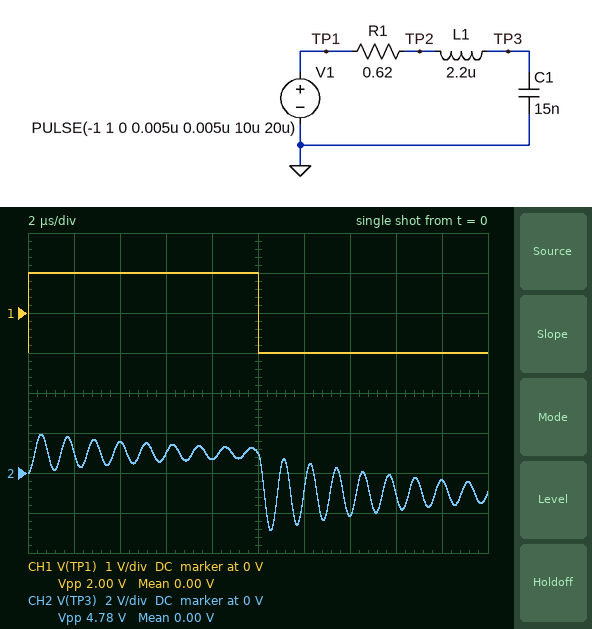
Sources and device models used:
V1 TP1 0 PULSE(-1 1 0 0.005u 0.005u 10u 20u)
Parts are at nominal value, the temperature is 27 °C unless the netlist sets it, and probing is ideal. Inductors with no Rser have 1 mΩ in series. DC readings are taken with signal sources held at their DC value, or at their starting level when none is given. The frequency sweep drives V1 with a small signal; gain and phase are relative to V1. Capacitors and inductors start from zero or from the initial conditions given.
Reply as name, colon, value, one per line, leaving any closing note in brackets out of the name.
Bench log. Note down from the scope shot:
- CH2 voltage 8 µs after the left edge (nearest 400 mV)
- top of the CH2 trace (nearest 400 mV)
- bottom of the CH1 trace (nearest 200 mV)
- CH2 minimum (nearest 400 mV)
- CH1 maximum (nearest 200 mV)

CH2 voltage 8 µs after the left edge: 800 mV
top of the CH2 trace: 2.0 V
bottom of the CH1 trace: -1.0 V
CH2 minimum: -2.8 V
CH1 maximum: 1.0 V
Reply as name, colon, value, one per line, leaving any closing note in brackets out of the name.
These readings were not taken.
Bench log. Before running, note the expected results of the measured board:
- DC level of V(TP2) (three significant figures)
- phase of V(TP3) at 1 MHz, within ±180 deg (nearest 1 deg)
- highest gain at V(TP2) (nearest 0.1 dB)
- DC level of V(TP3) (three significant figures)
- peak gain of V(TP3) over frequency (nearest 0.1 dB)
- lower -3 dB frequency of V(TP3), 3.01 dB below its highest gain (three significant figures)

DC level of V(TP2): -1.00 V
phase of V(TP3) at 1 MHz, within ±180 deg: -169 deg
highest gain at V(TP2): 0 dB
DC level of V(TP3): -1.00 V
peak gain of V(TP3) over frequency: 25.8 dB
lower -3 dB frequency of V(TP3), 3.01 dB below its highest gain: 853 kHz
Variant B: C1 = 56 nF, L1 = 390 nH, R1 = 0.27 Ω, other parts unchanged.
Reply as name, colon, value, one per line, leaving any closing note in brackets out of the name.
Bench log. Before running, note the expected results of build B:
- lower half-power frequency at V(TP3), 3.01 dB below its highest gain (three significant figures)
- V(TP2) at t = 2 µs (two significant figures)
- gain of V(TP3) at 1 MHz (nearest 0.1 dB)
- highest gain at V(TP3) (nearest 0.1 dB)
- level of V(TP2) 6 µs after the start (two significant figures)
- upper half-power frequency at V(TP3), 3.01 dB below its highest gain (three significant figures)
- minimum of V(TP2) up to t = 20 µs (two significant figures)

lower half-power frequency at V(TP3), 3.01 dB below its highest gain: 1.02 MHz
V(TP2) at t = 2 µs: 960 mV
gain of V(TP3) at 1 MHz: 15.5 dB
highest gain at V(TP3): 19.8 dB
level of V(TP2) 6 µs after the start: 1.0 V
upper half-power frequency at V(TP3), 3.01 dB below its highest gain: 1.13 MHz
minimum of V(TP2) up to t = 20 µs: -1.2 V
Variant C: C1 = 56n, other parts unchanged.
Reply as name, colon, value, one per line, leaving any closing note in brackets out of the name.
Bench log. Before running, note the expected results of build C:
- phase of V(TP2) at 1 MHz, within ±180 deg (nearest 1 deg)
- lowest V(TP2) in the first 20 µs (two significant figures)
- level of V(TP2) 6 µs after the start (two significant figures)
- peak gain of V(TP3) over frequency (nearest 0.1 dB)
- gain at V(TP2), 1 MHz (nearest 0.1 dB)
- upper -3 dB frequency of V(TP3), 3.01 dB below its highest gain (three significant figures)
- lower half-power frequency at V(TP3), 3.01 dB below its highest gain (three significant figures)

phase of V(TP2) at 1 MHz, within ±180 deg: 3 deg
lowest V(TP2) in the first 20 µs: -1.2 V
level of V(TP2) 6 µs after the start: 1.0 V
peak gain of V(TP3) over frequency: 20.1 dB
gain at V(TP2), 1 MHz: 0 dB
upper -3 dB frequency of V(TP3), 3.01 dB below its highest gain: 474 kHz
lower half-power frequency at V(TP3), 3.01 dB below its highest gain: 429 kHz
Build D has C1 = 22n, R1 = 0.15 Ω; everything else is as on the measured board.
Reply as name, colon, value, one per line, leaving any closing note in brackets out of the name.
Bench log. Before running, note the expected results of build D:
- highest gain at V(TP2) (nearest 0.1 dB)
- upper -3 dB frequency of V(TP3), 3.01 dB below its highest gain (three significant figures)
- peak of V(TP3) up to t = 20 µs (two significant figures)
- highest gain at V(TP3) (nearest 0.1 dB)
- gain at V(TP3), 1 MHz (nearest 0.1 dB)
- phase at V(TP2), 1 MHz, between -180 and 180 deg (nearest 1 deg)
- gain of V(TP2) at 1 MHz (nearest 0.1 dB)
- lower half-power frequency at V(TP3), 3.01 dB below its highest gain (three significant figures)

highest gain at V(TP2): 0 dB
upper -3 dB frequency of V(TP3), 3.01 dB below its highest gain: 729 kHz
peak of V(TP3) up to t = 20 µs: 2.0 V
highest gain at V(TP3): 36.4 dB
gain at V(TP3), 1 MHz: 0.8 dB
phase at V(TP2), 1 MHz, between -180 and 180 deg: 1 deg
gain of V(TP2) at 1 MHz: 0 dB
lower half-power frequency at V(TP3), 3.01 dB below its highest gain: 718 kHz
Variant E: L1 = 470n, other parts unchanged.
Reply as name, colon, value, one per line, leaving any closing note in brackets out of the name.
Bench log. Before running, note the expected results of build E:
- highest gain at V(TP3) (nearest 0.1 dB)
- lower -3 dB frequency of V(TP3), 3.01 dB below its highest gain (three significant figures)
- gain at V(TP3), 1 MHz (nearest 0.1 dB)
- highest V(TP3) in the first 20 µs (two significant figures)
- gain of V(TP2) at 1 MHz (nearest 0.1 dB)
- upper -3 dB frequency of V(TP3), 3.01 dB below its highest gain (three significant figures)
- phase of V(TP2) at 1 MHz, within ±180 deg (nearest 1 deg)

highest gain at V(TP3): 19.1 dB
lower -3 dB frequency of V(TP3), 3.01 dB below its highest gain: 1.78 MHz
gain at V(TP3), 1 MHz: 2.8 dB
highest V(TP3) in the first 20 µs: 1.8 V
gain of V(TP2) at 1 MHz: 0 dB
upper -3 dB frequency of V(TP3), 3.01 dB below its highest gain: 1.99 MHz
phase of V(TP2) at 1 MHz, within ±180 deg: -5 deg
